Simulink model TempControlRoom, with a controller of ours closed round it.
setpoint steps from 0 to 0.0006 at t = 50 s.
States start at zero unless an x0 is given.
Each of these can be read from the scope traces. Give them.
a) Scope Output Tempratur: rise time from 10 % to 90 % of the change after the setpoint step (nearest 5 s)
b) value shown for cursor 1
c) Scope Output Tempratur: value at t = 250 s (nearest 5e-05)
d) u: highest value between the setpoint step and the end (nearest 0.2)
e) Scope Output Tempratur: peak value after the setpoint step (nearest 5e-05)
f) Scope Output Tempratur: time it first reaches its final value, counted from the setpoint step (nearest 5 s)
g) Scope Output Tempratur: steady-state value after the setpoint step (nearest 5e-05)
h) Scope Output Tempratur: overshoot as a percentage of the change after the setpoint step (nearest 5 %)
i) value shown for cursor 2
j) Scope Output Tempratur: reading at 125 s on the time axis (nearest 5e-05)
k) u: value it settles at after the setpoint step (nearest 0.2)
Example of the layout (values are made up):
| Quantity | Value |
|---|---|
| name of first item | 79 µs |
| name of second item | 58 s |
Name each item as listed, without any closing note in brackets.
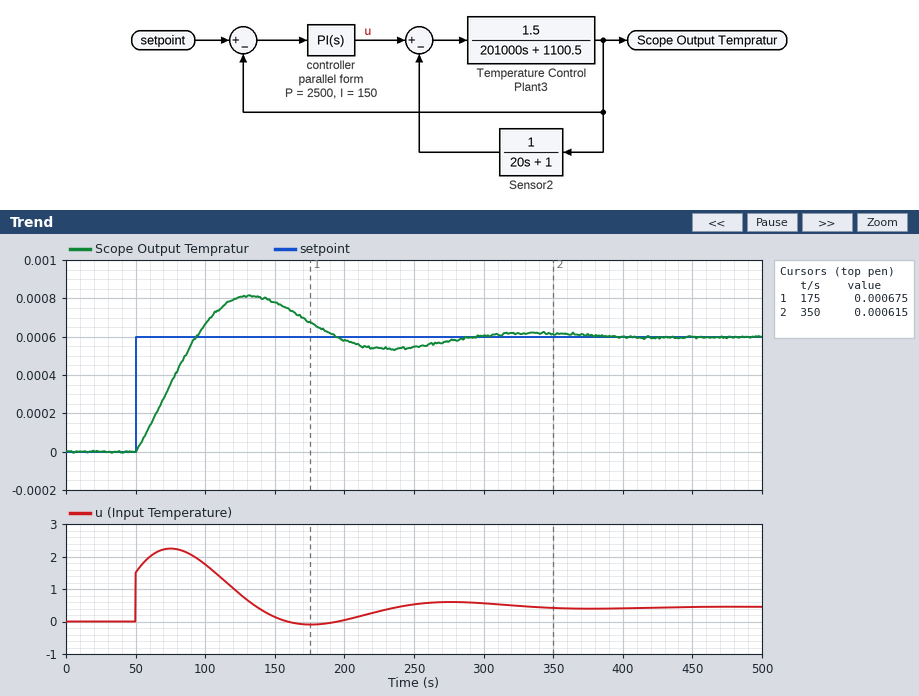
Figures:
| Quantity | Value |
|---|---|
| Scope Output Tempratur: rise time from 10 % to 90 % of the change after the setpoint step | 35 s |
| value shown for cursor 1 | 0.000675 |
| Scope Output Tempratur: value at t = 250 s | 0.00055 |
| u: highest value between the setpoint step and the end | 2.2 |
| Scope Output Tempratur: peak value after the setpoint step | 0.00080 |
| Scope Output Tempratur: time it first reaches its final value, counted from the setpoint step | 45 s |
| Scope Output Tempratur: steady-state value after the setpoint step | 0.00060 |
| Scope Output Tempratur: overshoot as a percentage of the change after the setpoint step | 35 % |
| value shown for cursor 2 | 0.000615 |
| Scope Output Tempratur: reading at 125 s on the time axis | 0.00080 |
| u: value it settles at after the setpoint step | 0.4 |
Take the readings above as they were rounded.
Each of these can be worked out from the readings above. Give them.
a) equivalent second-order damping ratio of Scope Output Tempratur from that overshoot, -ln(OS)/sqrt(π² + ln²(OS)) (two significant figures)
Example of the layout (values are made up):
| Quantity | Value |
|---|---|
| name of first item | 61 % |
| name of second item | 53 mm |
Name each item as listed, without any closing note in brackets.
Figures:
| Quantity | Value |
|---|---|
| equivalent second-order damping ratio of Scope Output Tempratur from that overshoot, -ln(OS)/sqrt(π² + ln²(OS)) | 0.32 |
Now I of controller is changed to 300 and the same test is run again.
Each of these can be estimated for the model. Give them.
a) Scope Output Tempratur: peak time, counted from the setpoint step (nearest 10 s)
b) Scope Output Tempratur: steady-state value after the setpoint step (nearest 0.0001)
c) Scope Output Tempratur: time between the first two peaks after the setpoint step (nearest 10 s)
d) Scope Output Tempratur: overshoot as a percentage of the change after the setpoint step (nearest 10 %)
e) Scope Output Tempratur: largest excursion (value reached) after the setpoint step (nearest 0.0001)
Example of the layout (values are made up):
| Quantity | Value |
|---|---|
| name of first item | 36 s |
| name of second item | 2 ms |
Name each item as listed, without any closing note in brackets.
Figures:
| Quantity | Value |
|---|---|
| Scope Output Tempratur: peak time, counted from the setpoint step | 60 s |
| Scope Output Tempratur: steady-state value after the setpoint step | 0.0006 |
| Scope Output Tempratur: time between the first two peaks after the setpoint step | 140 s |
| Scope Output Tempratur: overshoot as a percentage of the change after the setpoint step | 50 % |
| Scope Output Tempratur: largest excursion (value reached) after the setpoint step | 0.0009 |
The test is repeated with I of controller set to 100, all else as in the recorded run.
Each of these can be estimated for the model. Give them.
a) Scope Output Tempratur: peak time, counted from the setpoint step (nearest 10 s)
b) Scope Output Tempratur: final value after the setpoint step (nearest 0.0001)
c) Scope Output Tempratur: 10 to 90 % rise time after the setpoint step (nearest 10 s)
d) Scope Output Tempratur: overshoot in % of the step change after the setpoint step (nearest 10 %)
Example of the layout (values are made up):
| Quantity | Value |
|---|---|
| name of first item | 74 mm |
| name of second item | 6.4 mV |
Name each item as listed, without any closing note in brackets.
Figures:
| Quantity | Value |
|---|---|
| Scope Output Tempratur: peak time, counted from the setpoint step | 100 s |
| Scope Output Tempratur: final value after the setpoint step | 0.0006 |
| Scope Output Tempratur: 10 to 90 % rise time after the setpoint step | 40 s |
| Scope Output Tempratur: overshoot in % of the step change after the setpoint step | 30 % |
